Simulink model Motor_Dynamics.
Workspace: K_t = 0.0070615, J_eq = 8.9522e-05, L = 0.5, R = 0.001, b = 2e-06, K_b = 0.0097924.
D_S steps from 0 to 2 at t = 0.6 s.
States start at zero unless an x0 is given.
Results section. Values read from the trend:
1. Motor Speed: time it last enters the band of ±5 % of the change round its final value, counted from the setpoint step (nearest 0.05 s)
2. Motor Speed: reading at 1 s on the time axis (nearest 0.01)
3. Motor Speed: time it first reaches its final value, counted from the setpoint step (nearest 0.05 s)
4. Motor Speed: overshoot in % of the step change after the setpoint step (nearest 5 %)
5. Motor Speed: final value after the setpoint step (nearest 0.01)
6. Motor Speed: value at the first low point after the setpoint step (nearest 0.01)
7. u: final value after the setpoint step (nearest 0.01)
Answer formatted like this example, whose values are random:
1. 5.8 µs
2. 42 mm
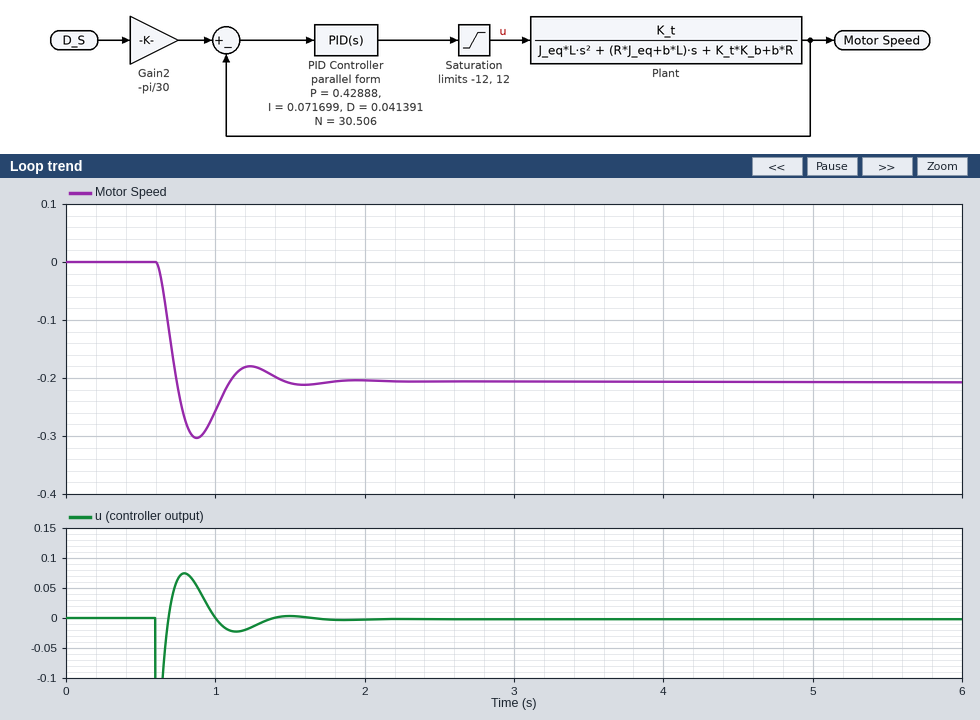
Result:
1. 0.80 s
2. -0.26
3. 0.15 s
4. 45 %
5. -0.21
6. -0.30
7. 0.00
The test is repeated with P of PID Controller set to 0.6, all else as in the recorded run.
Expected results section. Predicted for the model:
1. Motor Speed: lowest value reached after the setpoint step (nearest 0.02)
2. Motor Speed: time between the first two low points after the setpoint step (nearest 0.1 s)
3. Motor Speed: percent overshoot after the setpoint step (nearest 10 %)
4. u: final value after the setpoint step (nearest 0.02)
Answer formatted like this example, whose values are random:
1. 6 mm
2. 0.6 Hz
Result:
1. -0.32
2. 0.6 s
3. 50 %
4. 0.00
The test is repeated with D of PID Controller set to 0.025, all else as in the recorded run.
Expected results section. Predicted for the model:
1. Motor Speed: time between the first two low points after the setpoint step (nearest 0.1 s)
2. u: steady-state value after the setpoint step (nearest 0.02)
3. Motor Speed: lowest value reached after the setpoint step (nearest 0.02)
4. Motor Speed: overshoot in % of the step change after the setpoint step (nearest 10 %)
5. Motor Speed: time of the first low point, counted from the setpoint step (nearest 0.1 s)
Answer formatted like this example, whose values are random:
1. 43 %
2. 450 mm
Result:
1. 0.7 s
2. 0.00
3. -0.34
4. 60 %
5. 0.3 s
